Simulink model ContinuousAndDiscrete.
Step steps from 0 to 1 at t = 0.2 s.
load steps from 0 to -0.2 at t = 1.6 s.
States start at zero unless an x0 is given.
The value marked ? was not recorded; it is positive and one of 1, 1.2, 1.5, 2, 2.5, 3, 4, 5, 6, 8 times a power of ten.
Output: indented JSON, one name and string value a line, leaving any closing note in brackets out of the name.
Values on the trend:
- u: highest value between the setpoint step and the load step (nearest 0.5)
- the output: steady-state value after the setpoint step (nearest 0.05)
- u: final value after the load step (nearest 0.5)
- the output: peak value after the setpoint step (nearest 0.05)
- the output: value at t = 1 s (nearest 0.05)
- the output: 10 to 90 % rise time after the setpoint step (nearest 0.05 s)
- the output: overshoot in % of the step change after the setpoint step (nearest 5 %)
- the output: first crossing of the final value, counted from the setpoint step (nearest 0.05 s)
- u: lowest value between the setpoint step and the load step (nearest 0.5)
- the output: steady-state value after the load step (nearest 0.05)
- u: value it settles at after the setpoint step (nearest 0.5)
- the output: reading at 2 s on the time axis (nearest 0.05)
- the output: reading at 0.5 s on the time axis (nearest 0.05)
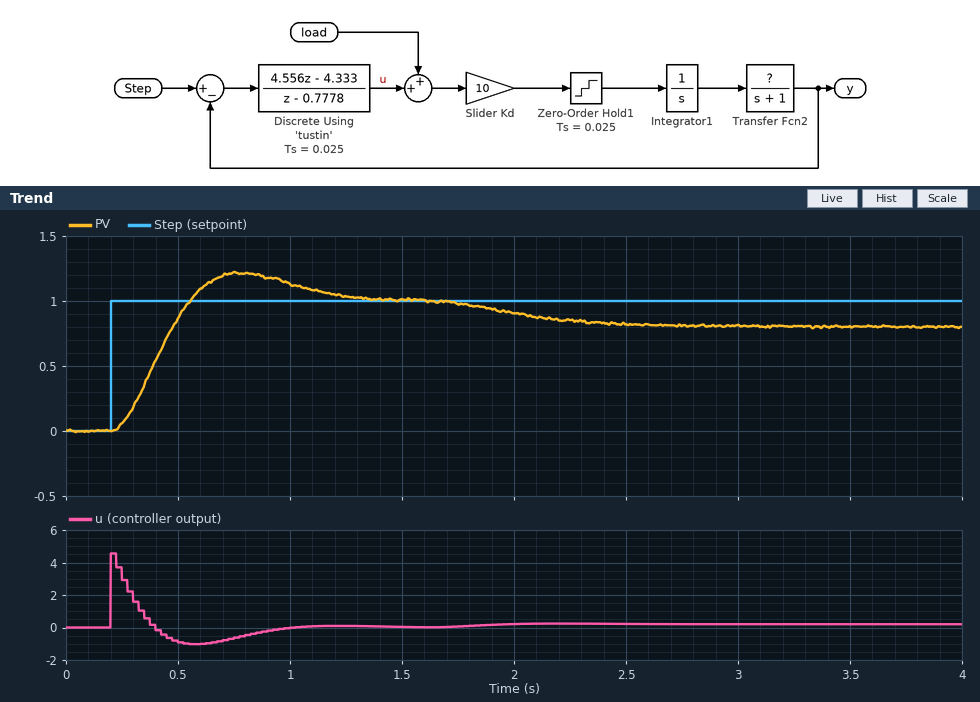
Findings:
{
  "u: highest value between the setpoint step and the load step": "4.5",
  "the output: steady-state value after the setpoint step": "1.00",
  "u: final value after the load step": "0.0",
  "the output: peak value after the setpoint step": "1.20",
  "the output: value at t = 1 s": "1.15",
  "the output: 10 to 90 % rise time after the setpoint step": "0.25 s",
  "the output: overshoot in % of the step change after the setpoint step": "20 %",
  "the output: first crossing of the final value, counted from the setpoint step": "0.35 s",
  "u: lowest value between the setpoint step and the load step": "-1.0",
  "the output: steady-state value after the load step": "0.80",
  "u: value it settles at after the setpoint step": "0.0",
  "the output: reading at 2 s on the time axis": "0.90",
  "the output: reading at 0.5 s on the time axis": "0.85"
}
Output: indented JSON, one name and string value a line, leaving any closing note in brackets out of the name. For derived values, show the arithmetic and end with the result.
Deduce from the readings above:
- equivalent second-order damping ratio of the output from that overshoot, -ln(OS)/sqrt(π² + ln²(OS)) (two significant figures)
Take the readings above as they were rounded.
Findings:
{
  "equivalent second-order damping ratio of the output from that overshoot, -ln(OS)/sqrt(π² + ln²(OS))": "ln(0.2) = -1.609; 1.609 / sqrt(9.870 + 2.590) = 0.46"
}
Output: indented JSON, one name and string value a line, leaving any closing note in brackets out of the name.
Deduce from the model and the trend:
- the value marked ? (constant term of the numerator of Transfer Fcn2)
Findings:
{
  "the value marked ?": "1"
}
